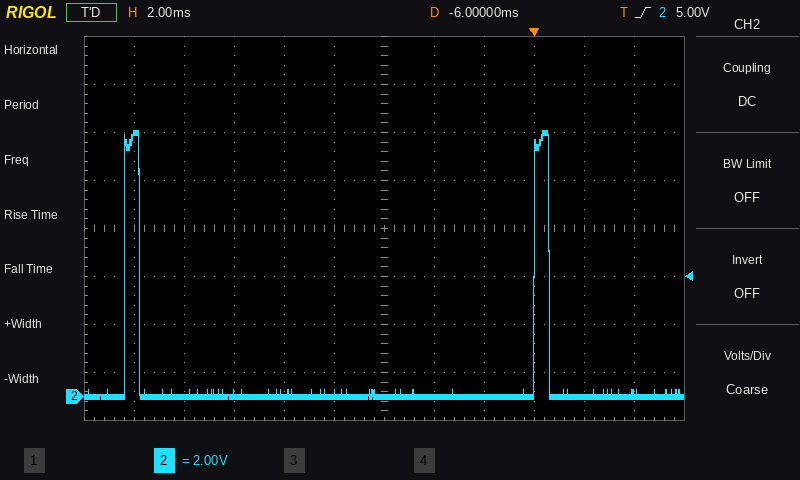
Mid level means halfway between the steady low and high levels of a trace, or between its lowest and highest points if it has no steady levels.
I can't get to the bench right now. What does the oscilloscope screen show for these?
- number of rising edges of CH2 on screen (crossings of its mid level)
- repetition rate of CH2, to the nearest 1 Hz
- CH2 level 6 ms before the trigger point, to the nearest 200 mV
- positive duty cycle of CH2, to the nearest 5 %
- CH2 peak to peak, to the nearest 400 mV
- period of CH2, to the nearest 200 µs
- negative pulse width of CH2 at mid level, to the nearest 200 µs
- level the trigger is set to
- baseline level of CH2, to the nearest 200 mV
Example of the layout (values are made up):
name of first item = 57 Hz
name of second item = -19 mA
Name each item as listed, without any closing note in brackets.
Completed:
number of rising edges of CH2 on screen = 2
repetition rate of CH2, to the nearest 1 Hz = 61 Hz
CH2 level 6 ms before the trigger point, to the nearest 200 mV = 0.0 V
positive duty cycle of CH2, to the nearest 5 % = 5 %
CH2 peak to peak, to the nearest 400 mV = 11.2 V
period of CH2, to the nearest 200 µs = 16.4 ms
negative pulse width of CH2 at mid level, to the nearest 200 µs = 15.8 ms
level the trigger is set to = 5.00 V
baseline level of CH2, to the nearest 200 mV = 0.0 V
